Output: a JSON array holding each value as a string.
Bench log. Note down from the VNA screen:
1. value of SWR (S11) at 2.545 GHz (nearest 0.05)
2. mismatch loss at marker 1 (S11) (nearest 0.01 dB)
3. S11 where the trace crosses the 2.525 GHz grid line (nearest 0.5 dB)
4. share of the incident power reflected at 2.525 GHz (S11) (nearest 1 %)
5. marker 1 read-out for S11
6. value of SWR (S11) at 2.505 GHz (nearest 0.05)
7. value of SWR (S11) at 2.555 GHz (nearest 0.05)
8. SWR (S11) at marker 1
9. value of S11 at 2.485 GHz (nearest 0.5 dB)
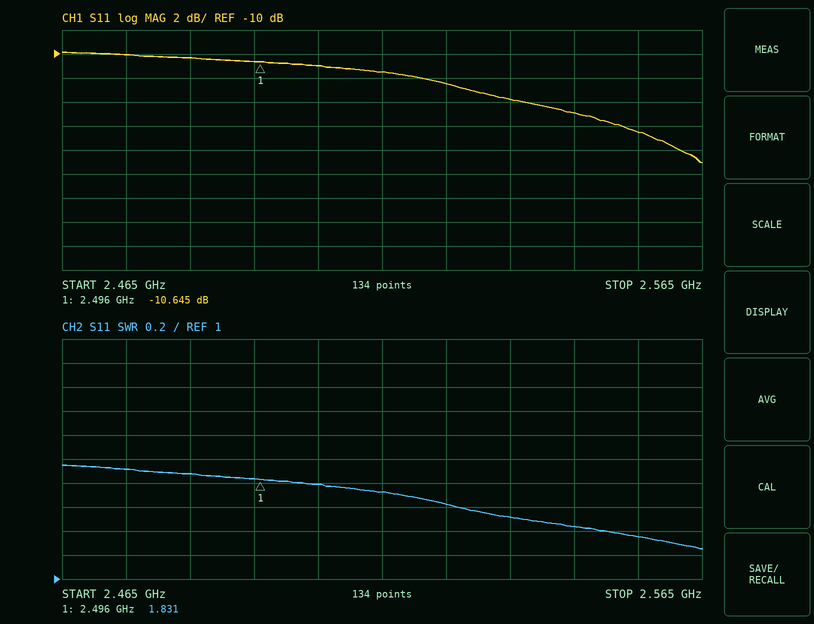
["1.45", "0.39 dB", "-12.5 dB", "6 %", "-10.645 dB", "1.80", "1.35", "1.831", "-10.5 dB"]
